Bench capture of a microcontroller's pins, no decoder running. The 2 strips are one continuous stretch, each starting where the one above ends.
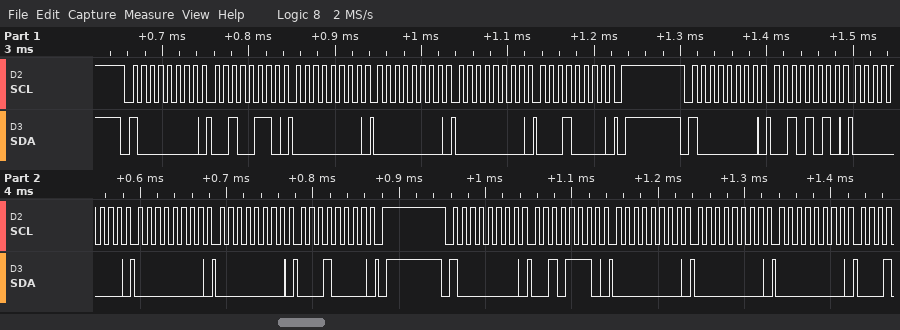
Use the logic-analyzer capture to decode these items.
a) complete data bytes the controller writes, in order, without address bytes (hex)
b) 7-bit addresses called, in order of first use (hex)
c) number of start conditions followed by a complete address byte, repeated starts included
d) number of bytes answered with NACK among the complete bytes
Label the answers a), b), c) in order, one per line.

a) 26 00 00 00 10 2A 00 00 00 10 2E 00 00 00
b) 0x40
c) 3
d) 0
